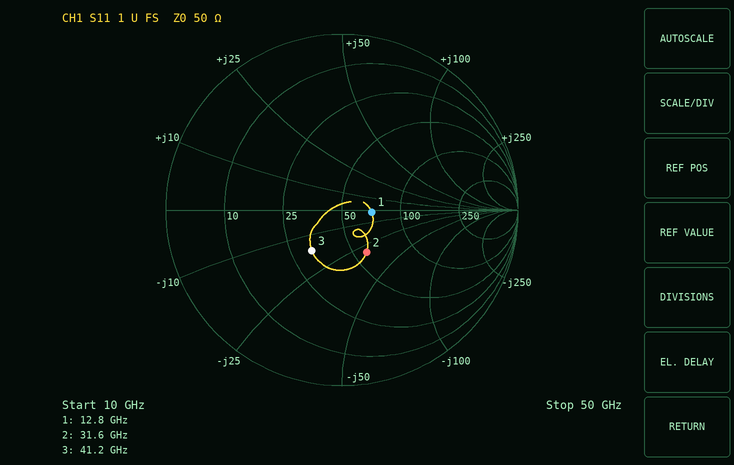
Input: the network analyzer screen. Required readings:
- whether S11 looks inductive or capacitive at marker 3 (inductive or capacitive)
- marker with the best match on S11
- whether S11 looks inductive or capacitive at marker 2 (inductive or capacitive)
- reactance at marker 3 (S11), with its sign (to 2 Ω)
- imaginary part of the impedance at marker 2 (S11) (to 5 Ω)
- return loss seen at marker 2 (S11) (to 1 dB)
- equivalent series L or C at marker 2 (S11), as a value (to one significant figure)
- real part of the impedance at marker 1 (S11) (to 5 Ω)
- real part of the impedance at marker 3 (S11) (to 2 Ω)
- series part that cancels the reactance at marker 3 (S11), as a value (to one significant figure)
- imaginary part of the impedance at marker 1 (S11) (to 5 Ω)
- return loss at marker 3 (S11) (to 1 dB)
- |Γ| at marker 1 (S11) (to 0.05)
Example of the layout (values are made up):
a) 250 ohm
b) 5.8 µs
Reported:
a) capacitive
b) marker 1
c) capacitive
d) -16 Ω
e) -30 Ω
f) 11 dB
g) 200 fF
h) 70 Ω
i) 32 Ω
j) 60 pH
k) 0 Ω
l) 11 dB
m) 0.15
